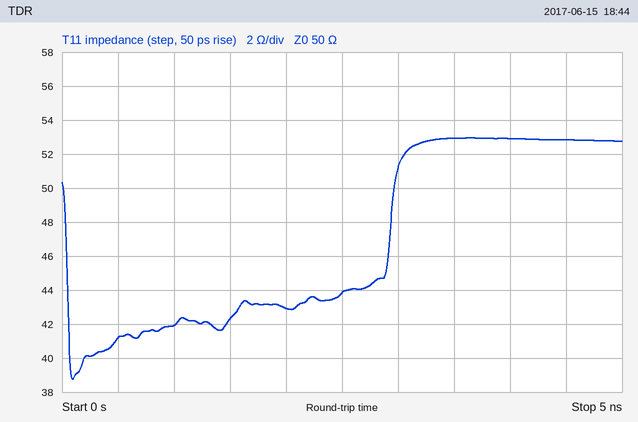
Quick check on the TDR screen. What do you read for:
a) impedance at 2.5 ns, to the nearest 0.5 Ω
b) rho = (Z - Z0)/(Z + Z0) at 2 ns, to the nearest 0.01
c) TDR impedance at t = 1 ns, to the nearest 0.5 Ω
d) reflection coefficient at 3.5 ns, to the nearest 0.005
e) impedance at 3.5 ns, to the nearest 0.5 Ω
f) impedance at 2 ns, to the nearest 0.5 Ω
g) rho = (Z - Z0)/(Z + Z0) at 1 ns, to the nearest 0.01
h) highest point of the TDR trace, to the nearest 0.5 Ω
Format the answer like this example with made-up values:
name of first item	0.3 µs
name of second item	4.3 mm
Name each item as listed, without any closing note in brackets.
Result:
impedance at 2.5 ns, to the nearest 0.5 Ω	44.0 Ω
rho = (Z - Z0)/(Z + Z0) at 2 ns, to the nearest 0.01	-0.08
TDR impedance at t = 1 ns, to the nearest 0.5 Ω	42.0 Ω
reflection coefficient at 3.5 ns, to the nearest 0.005	+0.030
impedance at 3.5 ns, to the nearest 0.5 Ω	53.0 Ω
impedance at 2 ns, to the nearest 0.5 Ω	43.0 Ω
rho = (Z - Z0)/(Z + Z0) at 1 ns, to the nearest 0.01	-0.09
highest point of the TDR trace, to the nearest 0.5 Ω	53.0 Ω
